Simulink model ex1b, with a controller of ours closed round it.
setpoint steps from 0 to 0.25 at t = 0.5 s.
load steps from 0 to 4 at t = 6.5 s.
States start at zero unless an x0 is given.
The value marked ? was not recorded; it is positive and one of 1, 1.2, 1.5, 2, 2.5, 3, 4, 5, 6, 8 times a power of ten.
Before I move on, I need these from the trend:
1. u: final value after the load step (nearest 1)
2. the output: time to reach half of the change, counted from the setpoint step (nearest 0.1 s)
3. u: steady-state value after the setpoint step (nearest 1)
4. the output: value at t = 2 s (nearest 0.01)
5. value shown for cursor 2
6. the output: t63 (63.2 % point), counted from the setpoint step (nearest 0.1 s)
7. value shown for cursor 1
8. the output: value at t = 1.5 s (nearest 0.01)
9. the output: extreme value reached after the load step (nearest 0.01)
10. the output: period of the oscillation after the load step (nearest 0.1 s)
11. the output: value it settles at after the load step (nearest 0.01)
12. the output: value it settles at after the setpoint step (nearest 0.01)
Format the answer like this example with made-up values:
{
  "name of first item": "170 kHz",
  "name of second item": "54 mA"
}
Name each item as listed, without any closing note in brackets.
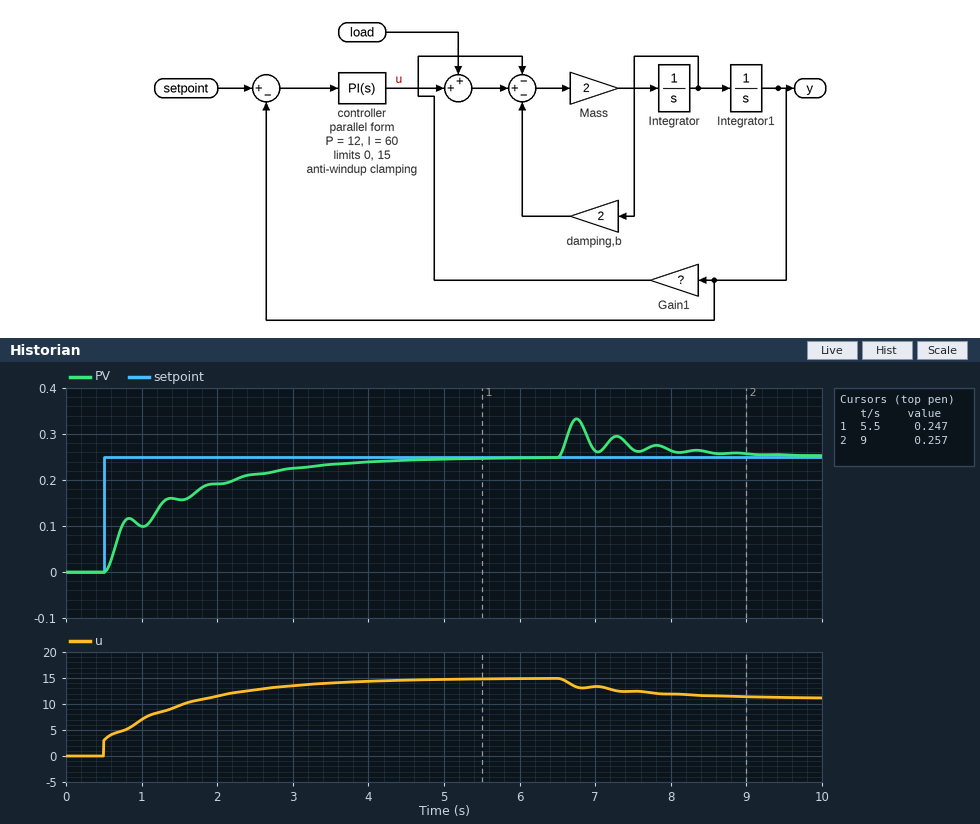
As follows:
{
  "u: final value after the load step": "11",
  "the output: time to reach half of the change, counted from the setpoint step": "0.7 s",
  "u: steady-state value after the setpoint step": "15",
  "the output: value at t = 2 s": "0.19",
  "value shown for cursor 2": "0.257",
  "the output: t63 (63.2 % point), counted from the setpoint step": "0.8 s",
  "value shown for cursor 1": "0.247",
  "the output: value at t = 1.5 s": "0.16",
  "the output: extreme value reached after the load step": "0.33",
  "the output: period of the oscillation after the load step": "0.5 s",
  "the output: value it settles at after the load step": "0.25",
  "the output: value it settles at after the setpoint step": "0.25"
}
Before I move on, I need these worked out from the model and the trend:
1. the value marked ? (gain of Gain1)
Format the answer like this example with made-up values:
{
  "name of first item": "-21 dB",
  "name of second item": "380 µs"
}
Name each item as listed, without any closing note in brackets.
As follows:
{
  "the value marked ?": "60"
}
